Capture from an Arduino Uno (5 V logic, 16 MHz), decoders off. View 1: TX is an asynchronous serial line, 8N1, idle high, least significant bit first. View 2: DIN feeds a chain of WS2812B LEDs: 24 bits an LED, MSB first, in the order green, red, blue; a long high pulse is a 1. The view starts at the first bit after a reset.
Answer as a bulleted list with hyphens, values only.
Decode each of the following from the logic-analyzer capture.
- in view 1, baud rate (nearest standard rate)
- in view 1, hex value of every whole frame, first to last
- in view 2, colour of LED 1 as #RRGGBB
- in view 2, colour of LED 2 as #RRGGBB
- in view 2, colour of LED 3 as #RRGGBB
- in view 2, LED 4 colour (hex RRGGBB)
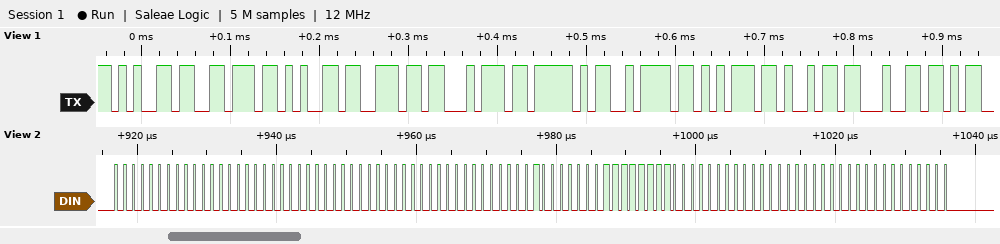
- 115200 baud
- 0x65 0x76 0x65 0x6E 0x74 0x5F 0x7A 0x75 0x69 0x64
- #000000
- #000000
- #FF8000
- #000000
